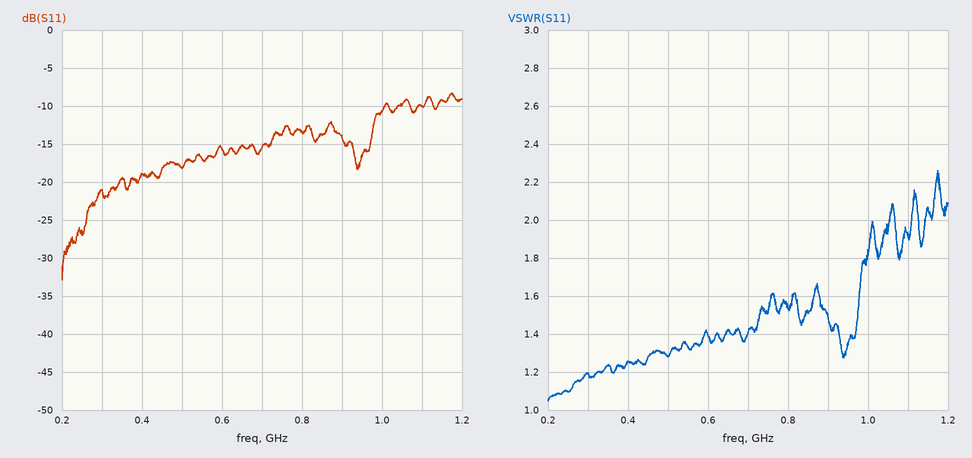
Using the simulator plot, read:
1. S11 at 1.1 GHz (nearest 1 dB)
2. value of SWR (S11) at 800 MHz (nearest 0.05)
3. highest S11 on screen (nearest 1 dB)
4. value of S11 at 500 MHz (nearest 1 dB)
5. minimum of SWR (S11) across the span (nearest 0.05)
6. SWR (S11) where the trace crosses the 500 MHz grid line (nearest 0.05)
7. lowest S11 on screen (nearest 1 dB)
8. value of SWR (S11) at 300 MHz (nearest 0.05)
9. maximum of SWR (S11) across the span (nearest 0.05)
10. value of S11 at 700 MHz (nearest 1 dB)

-10 dB
1.55
-8 dB
-18 dB
1.05
1.30
-33 dB
1.20
2.25
-15 dB
